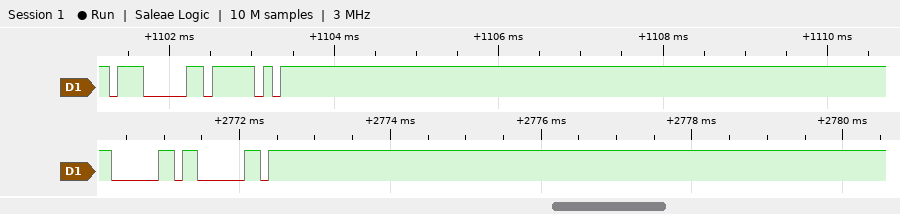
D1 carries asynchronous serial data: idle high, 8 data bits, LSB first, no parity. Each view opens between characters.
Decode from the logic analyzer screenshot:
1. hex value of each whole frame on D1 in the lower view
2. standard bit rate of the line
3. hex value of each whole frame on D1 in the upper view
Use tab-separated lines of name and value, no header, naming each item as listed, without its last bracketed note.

hex value of each whole frame on D1 in the lower view	60, 60
standard bit rate of the line	9600 baud
hex value of each whole frame on D1 in the upper view	07, 5F
